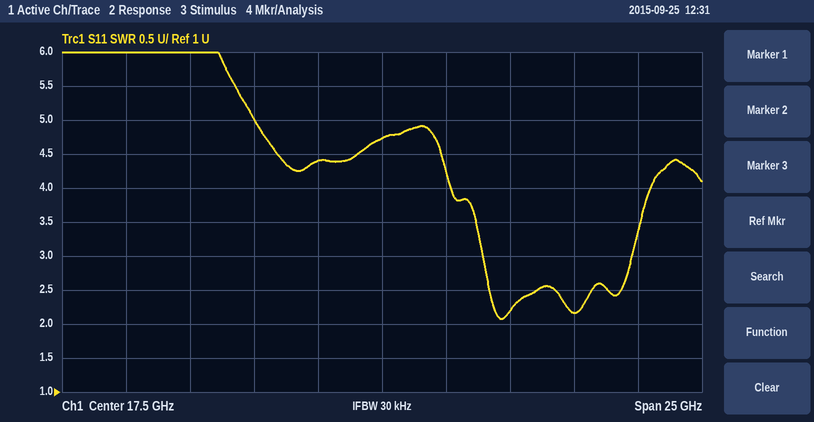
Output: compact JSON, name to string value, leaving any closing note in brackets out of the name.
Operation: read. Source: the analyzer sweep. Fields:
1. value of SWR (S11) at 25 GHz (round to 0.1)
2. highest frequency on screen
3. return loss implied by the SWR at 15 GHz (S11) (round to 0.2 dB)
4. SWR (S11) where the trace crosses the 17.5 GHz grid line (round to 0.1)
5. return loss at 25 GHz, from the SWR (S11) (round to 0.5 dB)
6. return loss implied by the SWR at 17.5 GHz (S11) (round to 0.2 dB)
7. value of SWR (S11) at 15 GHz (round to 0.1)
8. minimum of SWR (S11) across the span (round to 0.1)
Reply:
{"value of SWR (S11) at 25 GHz": "2.2", "highest frequency on screen": "30 GHz", "return loss implied by the SWR at 15 GHz (S11)": "4.0 dB", "SWR (S11) where the trace crosses the 17.5 GHz grid line": "4.7", "return loss at 25 GHz, from the SWR (S11)": "8.5 dB", "return loss implied by the SWR at 17.5 GHz (S11)": "3.8 dB", "value of SWR (S11) at 15 GHz": "4.4", "minimum of SWR (S11) across the span": "2.1"}
